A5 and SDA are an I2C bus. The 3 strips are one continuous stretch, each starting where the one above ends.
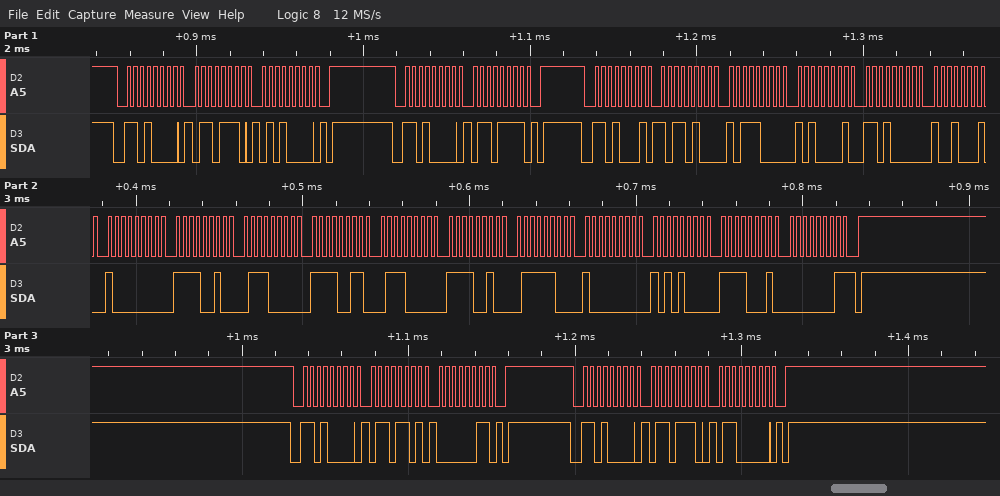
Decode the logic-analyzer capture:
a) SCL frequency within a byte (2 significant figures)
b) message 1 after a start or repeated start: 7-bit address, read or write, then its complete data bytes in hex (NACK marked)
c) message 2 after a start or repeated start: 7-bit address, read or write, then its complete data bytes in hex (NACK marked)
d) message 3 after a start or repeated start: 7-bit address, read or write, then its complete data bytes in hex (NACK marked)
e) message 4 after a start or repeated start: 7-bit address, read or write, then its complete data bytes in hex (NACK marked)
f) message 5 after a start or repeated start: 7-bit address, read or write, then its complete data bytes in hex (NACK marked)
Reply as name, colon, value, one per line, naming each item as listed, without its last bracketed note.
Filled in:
SCL frequency within a byte: 250 kHz
message 1 after a start or repeated start: 7-bit address, read or write, then its complete data bytes in hex: 0x68 write: 6E 50
message 2 after a start or repeated start: 7-bit address, read or write, then its complete data bytes in hex: 0x68 write: 6F
message 3 after a start or repeated start: 7-bit address, read or write, then its complete data bytes in hex: 0x68 read: B4 B8 A1 D0 91 80 F2 70 F3 70 F2 7C 80 A8 F1 01 NACK
message 4 after a start or repeated start: 7-bit address, read or write, then its complete data bytes in hex: 0x68 write: 6D 03
message 5 after a start or repeated start: 7-bit address, read or write, then its complete data bytes in hex: 0x68 write: 6E 60
